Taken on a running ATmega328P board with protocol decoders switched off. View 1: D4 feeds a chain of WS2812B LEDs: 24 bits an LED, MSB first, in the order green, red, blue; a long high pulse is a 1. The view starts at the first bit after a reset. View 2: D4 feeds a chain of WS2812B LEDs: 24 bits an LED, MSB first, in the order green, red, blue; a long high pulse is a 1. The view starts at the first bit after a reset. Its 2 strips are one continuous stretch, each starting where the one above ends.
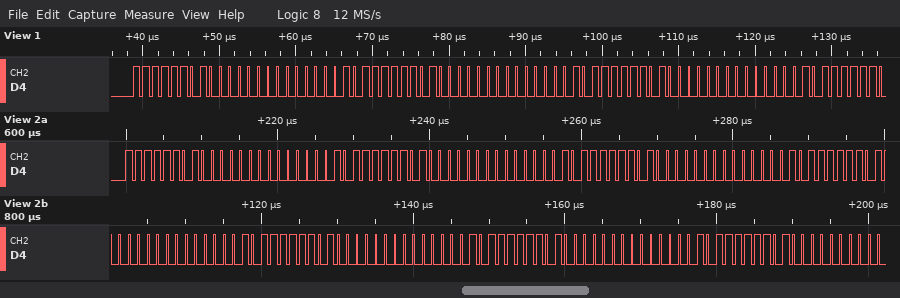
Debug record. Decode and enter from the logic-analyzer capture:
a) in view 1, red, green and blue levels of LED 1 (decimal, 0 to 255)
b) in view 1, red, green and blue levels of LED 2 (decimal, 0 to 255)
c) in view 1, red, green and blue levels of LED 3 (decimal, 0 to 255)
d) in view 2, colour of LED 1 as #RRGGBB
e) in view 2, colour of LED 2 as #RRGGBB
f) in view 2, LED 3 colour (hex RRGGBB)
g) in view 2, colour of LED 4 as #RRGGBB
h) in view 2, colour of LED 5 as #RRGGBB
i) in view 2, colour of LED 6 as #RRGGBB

0, 253, 2
0, 253, 2
0, 253, 2
#00FD02
#00FD02
#00FD02
#00FD02
#00FD02
#00FD02
